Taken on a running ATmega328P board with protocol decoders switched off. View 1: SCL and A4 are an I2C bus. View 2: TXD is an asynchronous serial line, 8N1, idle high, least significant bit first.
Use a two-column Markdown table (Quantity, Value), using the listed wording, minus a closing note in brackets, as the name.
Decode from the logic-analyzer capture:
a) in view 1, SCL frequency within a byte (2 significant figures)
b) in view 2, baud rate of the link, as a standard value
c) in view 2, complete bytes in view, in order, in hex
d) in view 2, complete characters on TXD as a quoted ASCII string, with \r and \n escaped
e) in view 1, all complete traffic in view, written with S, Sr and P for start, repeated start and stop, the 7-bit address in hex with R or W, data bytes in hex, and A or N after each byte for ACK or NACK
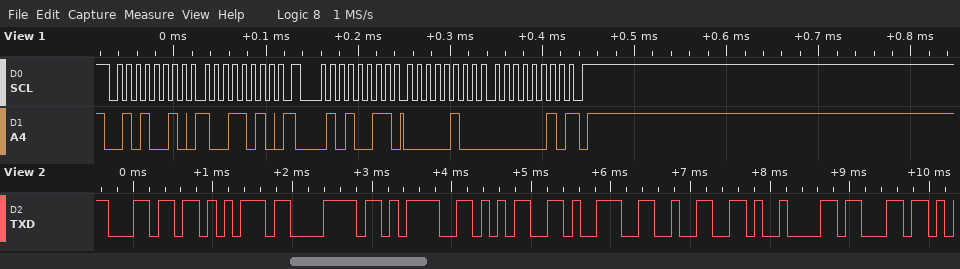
| Quantity | Value |
|---|---|
| in view 1, SCL frequency within a byte | 100 kHz |
| in view 2, baud rate of the link, as a standard value | 9600 baud |
| in view 2, complete bytes in view, in order, in hex | 6C 75 78 3D 35 39 32 09 63 |
| in view 2, complete characters on TXD as a quoted ASCII string, with \r and \n escaped | "lux=592\tc" |
| in view 1, all complete traffic in view, written with S, Sr and P for start, repeated start and stop, the 7-bit address in hex with R or W, data bytes in hex, and A or N after each byte for ACK or NACK | S 29W A 9A A Sr 29R A 04 A 02 N P |
